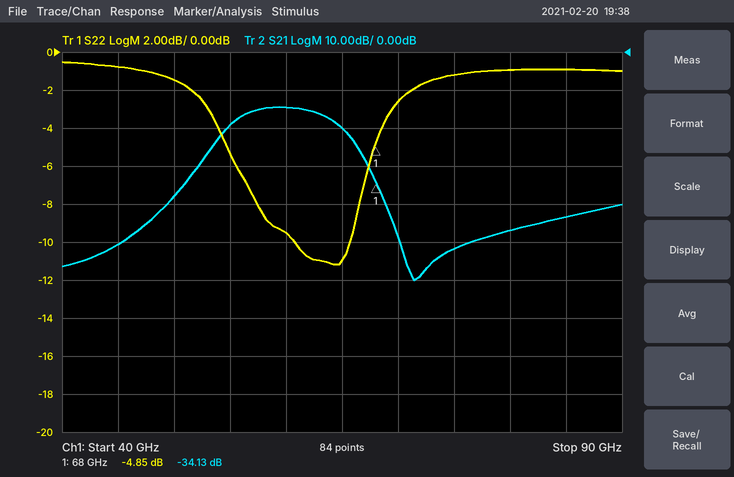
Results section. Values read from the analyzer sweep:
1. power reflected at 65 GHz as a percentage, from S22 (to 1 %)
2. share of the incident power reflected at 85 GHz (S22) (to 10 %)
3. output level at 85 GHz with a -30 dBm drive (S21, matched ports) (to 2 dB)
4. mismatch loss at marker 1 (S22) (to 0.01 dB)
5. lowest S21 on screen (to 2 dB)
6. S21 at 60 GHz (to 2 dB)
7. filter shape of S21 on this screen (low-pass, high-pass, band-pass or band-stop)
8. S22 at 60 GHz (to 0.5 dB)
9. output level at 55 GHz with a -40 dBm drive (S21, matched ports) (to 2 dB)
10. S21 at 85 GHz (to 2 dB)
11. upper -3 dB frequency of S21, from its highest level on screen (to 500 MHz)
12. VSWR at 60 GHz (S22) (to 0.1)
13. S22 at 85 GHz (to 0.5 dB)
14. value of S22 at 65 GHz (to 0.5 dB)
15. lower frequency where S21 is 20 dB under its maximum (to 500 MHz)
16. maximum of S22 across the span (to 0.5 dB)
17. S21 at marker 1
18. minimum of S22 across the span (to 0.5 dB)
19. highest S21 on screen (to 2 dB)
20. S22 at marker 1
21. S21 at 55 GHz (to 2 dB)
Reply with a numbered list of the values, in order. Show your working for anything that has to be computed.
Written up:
1. 10^(-11/10) ≈ 8 %
2. 10^(-1/10) ≈ 79.4 %, so 80 % to the nearest 10 %
3. -30 dBm + (-44 dB) = -74 dBm
4. −10 log10(1 − 10^(-4.85/10)) ≈ 1.72 dB
5. -60 dB
6. -14 dB
7. band-pass
8. -9.5 dB
9. -40 dBm + (-20 dB) = -60 dBm
10. -44 dB
11. 64.0 GHz
12. |Γ| = 10^(-9.5/20) = 0.3350; VSWR = (1 + 0.3350)/(1 − 0.3350) ≈ 2.0
13. -1.0 dB
14. -11.0 dB
15. 51.0 GHz
16. -0.5 dB
17. -34.13 dB
18. -11.0 dB
19. -14 dB
20. -4.85 dB
21. -20 dB
